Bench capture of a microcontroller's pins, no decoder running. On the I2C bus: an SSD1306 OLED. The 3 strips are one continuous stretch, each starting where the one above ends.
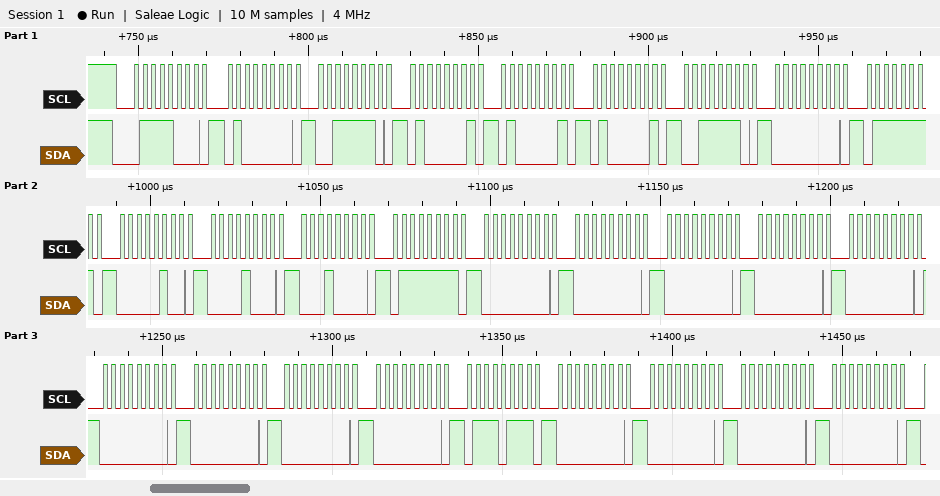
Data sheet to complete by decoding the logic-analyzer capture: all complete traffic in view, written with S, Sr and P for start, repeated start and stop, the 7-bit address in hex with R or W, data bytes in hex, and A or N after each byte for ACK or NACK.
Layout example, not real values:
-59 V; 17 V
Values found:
S 3CW A 40 A 3E A 41 A 41 A 41 A 3E A 00 A 7F A 04 A 08 A 10 A 7F A 00 A 00 A 00 A 00 A 00 A 00 A 00 A 00 A 00 A 77 A 00 A 00 A 00 A 00 A
